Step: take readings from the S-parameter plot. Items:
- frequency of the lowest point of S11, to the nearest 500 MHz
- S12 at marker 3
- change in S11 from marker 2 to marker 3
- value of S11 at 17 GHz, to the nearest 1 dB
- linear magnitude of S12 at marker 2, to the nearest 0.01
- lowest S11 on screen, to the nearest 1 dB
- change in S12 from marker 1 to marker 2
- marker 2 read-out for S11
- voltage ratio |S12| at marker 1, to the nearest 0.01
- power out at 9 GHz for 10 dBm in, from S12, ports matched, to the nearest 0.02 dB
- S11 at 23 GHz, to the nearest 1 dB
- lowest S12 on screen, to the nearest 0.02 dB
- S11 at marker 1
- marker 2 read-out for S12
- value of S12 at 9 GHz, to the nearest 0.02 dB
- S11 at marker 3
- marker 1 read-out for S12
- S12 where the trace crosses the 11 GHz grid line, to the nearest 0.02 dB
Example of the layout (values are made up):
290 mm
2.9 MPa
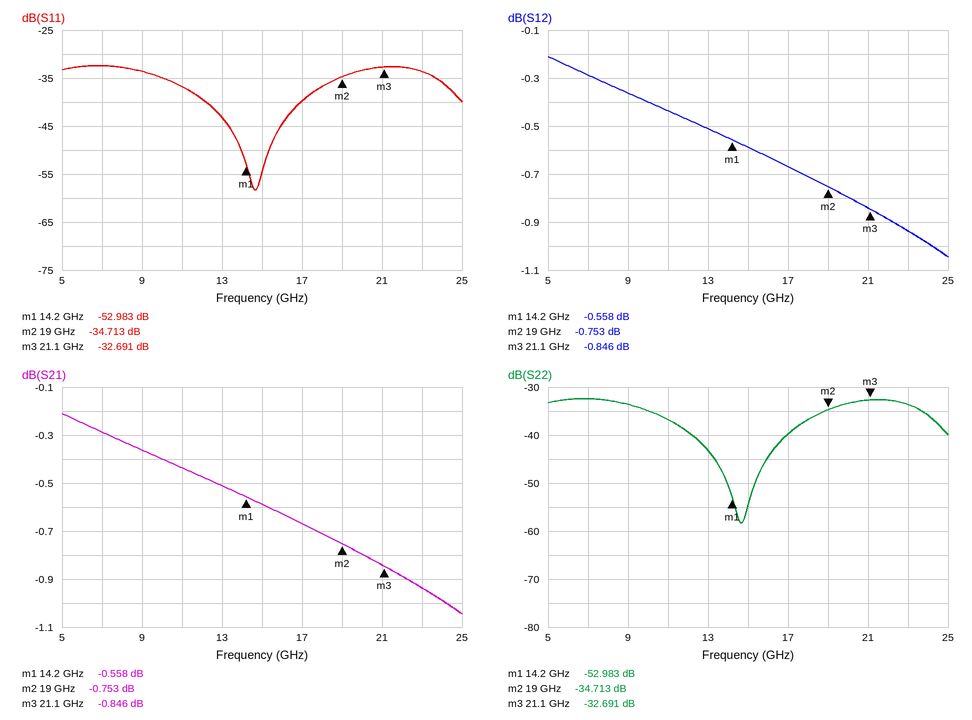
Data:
14.5 GHz
-0.846 dB
2.022 dB
-40 dB
0.92
-58 dB
-0.195 dB
-34.713 dB
0.94
9.64 dBm
-34 dB
-1.04 dB
-52.983 dB
-0.753 dB
-0.36 dB
-32.691 dB
-0.558 dB
-0.44 dB
